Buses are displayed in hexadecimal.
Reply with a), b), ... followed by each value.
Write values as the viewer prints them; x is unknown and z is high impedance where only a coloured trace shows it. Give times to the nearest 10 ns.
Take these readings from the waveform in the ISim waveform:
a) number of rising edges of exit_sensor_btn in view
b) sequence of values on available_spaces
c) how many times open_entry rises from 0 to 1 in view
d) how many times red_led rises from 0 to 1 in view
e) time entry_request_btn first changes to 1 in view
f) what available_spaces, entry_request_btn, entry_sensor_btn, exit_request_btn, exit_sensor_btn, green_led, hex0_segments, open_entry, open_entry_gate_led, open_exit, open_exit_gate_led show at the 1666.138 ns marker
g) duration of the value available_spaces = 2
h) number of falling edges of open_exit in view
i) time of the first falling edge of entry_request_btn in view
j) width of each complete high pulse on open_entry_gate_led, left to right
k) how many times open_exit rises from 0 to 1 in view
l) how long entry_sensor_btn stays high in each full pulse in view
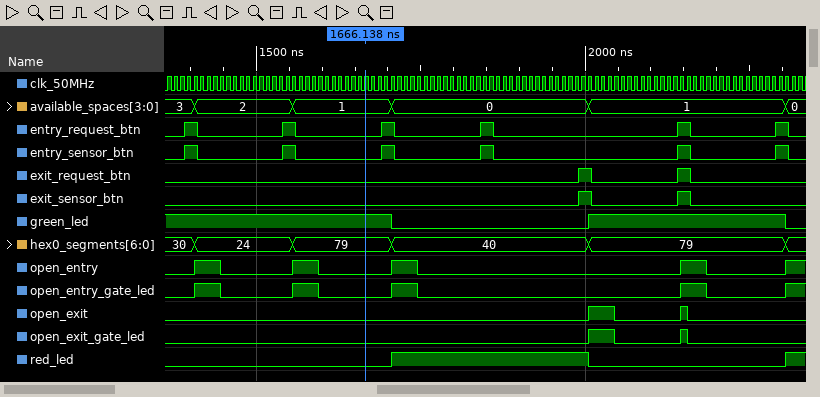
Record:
a) 2
b) 3, 2, 1, 0, 1, 0
c) 5
d) 2
e) 1390 ns
f) available_spaces=1, entry_request_btn=0, entry_sensor_btn=0, exit_request_btn=0, exit_sensor_btn=0, green_led=1, hex0_segments=79, open_entry=0, open_entry_gate_led=0, open_exit=0, open_exit_gate_led=0
g) 150 ns
h) 2
i) 1410 ns
j) 40 ns, 40 ns, 40 ns, 40 ns
k) 2
l) 20 ns, 20 ns, 20 ns, 20 ns, 20 ns, 20 ns
